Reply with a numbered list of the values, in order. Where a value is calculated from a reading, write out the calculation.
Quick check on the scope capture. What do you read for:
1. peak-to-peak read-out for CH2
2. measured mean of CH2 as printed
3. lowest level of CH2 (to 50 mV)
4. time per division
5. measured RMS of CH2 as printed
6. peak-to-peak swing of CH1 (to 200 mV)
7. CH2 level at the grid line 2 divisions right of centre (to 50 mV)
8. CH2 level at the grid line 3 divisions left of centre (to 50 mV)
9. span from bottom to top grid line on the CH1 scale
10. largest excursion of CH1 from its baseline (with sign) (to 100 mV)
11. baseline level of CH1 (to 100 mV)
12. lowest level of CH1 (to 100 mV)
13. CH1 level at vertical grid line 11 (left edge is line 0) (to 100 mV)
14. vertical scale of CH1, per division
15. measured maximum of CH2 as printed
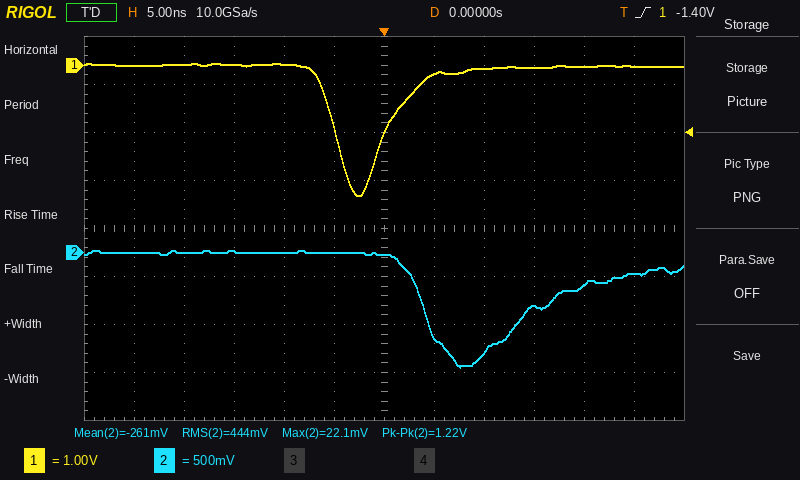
1. 1.22 V
2. -261 mV
3. -1.20 V
4. 5 ns
5. 444 mV
6. 2.8 V
7. -1.05 V
8. 0 mV
9. 8 V
10. -2.7 V − (0.0 V) = -2.7 V
11. 0.0 V
12. -2.7 V
13. 0.0 V
14. 1 V
15. 22.1 mV
